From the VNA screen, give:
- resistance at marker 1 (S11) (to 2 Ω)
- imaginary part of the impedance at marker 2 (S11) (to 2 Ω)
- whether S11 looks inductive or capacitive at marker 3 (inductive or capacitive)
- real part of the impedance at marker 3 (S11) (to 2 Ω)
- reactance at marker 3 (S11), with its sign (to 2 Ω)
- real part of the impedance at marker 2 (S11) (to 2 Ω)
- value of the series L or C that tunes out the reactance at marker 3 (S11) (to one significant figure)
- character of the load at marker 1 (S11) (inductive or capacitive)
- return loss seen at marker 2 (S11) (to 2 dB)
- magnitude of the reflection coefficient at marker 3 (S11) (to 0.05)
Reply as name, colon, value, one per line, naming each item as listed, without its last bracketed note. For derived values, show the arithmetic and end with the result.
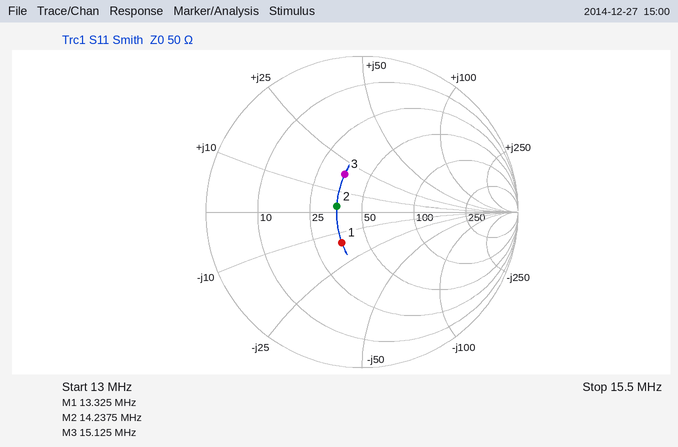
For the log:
resistance at marker 1 (S11): 36 Ω
imaginary part of the impedance at marker 2 (S11): +2 Ω
whether S11 looks inductive or capacitive at marker 3: inductive
real part of the impedance at marker 3 (S11): 36 Ω
reactance at marker 3 (S11), with its sign: +18 Ω
real part of the impedance at marker 2 (S11): 36 Ω
value of the series L or C that tunes out the reactance at marker 3 (S11): C = 1/(2π × 15.125 MHz × 18 Ω) ≈ 585 pF, so 600 pF to one significant figure
character of the load at marker 1 (S11): capacitive
return loss seen at marker 2 (S11): 16 dB
magnitude of the reflection coefficient at marker 3 (S11): 0.25
